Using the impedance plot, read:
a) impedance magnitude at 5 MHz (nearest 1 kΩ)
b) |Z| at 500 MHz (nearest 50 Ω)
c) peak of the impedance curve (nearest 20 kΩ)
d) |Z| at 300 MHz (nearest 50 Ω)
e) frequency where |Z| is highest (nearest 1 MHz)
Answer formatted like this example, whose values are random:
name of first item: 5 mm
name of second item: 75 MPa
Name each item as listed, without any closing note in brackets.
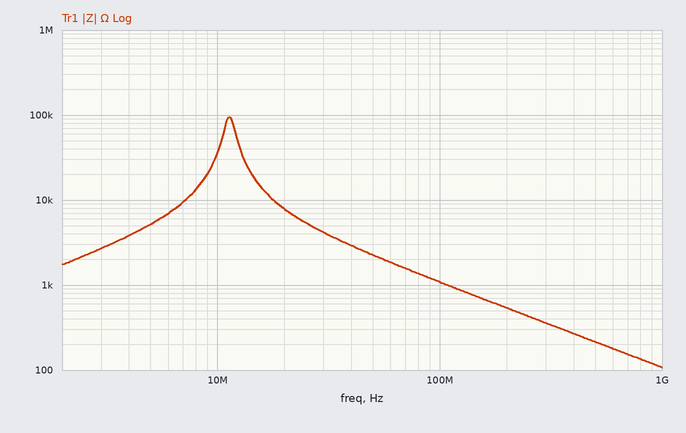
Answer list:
impedance magnitude at 5 MHz: 5 kΩ
|Z| at 500 MHz: 200 Ω
peak of the impedance curve: 100 kΩ
|Z| at 300 MHz: 350 Ω
frequency where |Z| is highest: 11 MHz
